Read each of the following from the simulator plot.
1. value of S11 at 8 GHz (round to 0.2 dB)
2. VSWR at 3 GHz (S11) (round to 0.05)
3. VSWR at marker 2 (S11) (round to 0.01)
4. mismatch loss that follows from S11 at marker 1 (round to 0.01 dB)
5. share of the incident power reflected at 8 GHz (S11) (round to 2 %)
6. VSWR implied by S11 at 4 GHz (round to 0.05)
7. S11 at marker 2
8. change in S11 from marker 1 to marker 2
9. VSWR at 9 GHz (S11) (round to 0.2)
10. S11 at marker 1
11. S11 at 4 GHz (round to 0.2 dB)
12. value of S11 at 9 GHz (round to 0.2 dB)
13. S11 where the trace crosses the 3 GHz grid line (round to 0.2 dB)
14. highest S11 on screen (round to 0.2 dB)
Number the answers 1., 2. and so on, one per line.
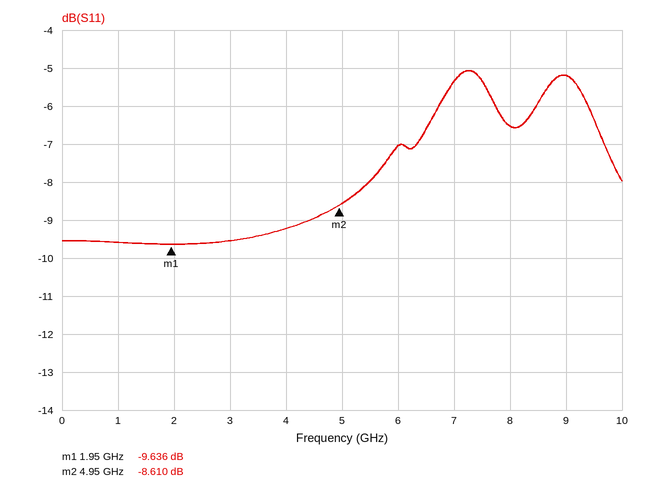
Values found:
1. -6.6 dB
2. 2.00
3. 2.18
4. 0.50 dB
5. 22 %
6. 2.05
7. -8.610 dB
8. 1.026 dB
9. 3.4
10. -9.636 dB
11. -9.2 dB
12. -5.2 dB
13. -9.6 dB
14. -5.0 dB
